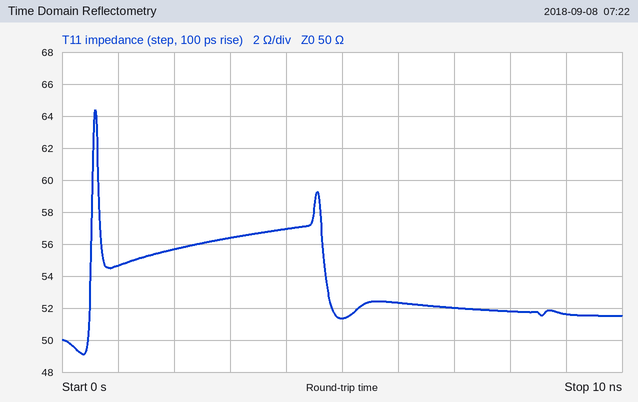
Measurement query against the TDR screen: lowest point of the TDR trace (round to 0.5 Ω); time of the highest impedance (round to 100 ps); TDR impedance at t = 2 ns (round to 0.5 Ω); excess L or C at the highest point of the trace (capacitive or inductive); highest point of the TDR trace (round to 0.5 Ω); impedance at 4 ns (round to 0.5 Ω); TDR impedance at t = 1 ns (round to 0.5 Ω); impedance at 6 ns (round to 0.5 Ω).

49.0 Ω
600 ps
55.5 Ω
inductive
64.5 Ω
57.0 Ω
54.5 Ω
52.5 Ω
